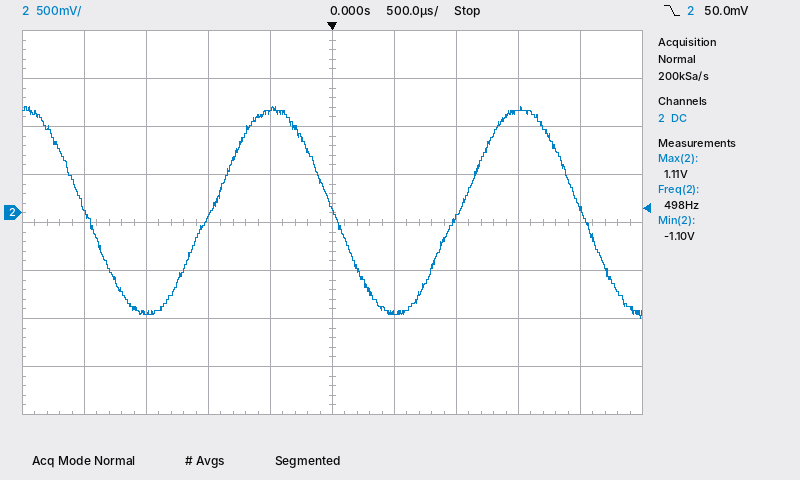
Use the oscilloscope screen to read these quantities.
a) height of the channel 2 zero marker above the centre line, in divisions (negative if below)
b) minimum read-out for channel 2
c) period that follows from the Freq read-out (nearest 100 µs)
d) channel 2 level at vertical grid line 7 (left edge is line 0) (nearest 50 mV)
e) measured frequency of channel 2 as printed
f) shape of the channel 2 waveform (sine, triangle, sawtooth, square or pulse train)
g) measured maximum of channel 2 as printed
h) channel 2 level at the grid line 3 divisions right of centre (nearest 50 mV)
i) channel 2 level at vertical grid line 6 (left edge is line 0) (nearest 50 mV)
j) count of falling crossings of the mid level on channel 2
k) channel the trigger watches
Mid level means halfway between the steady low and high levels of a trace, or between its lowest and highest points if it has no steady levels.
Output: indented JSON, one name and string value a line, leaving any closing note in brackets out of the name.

{
  "height of the channel 2 zero marker above the centre line, in divisions": "+0.2 div",
  "minimum read-out for channel 2": "-1.10 V",
  "period that follows from the Freq read-out": "2.0 ms",
  "channel 2 level at vertical grid line 7 (left edge is line 0)": "-50 mV",
  "measured frequency of channel 2 as printed": "498 Hz",
  "shape of the channel 2 waveform": "sine",
  "measured maximum of channel 2 as printed": "1.11 V",
  "channel 2 level at the grid line 3 divisions right of centre": "1.10 V",
  "channel 2 level at vertical grid line 6 (left edge is line 0)": "-1.05 V",
  "count of falling crossings of the mid level on channel 2": "3",
  "channel the trigger watches": "channel 2"
}
